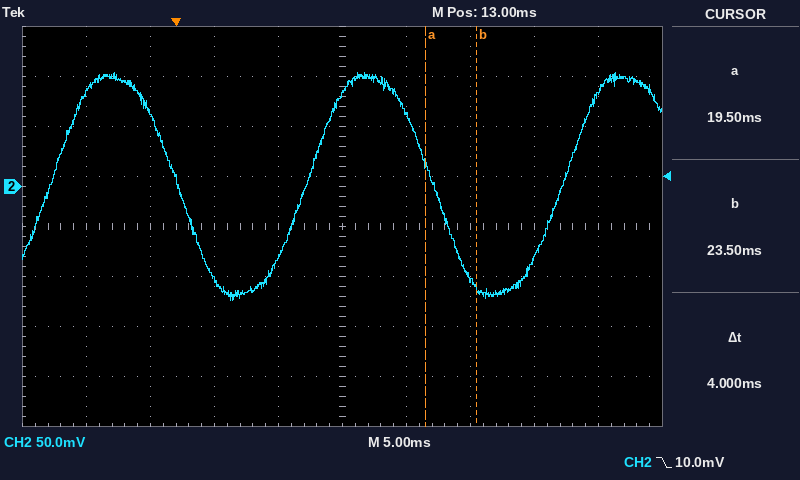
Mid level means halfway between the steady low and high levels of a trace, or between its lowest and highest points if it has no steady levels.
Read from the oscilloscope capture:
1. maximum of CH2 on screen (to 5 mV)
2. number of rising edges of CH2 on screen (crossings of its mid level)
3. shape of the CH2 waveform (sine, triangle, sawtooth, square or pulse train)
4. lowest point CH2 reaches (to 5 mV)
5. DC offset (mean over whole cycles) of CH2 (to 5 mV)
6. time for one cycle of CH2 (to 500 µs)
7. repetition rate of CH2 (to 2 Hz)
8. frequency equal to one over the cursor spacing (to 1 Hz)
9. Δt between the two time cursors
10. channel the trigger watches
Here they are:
115 mV
3
sine
-115 mV
0 mV
20.0 ms
50 Hz
250 Hz
4 ms
CH2
